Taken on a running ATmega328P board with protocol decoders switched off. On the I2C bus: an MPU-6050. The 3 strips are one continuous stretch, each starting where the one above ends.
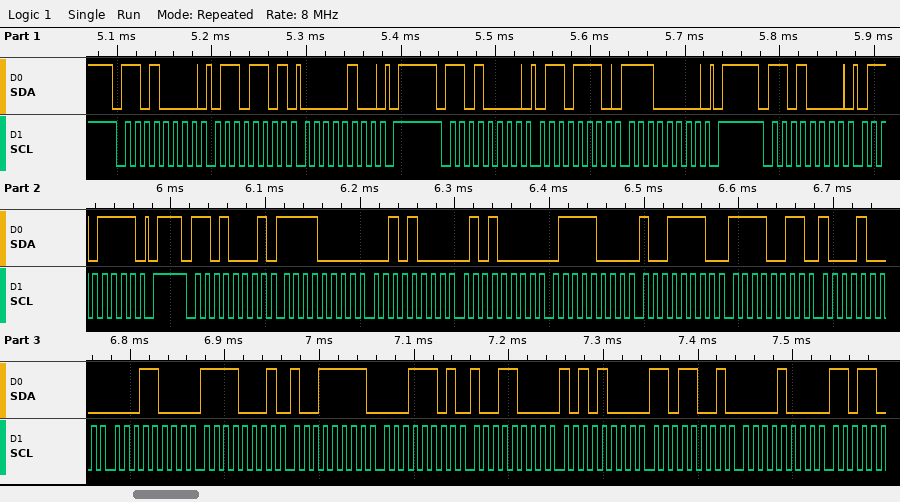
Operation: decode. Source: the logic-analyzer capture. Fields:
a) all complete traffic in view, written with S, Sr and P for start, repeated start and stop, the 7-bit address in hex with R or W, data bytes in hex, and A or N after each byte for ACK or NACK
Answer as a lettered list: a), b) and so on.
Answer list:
a) S 68W A 6D A 04 A P S 68W A 6E A E0 A P S 68W A 6F A P S 68R A F0 A 28 A 50 A 78 A 9E A F3 A 88 A 18 A F1 A 9F A 1D A 98 A A8 A D9 A 08 A
